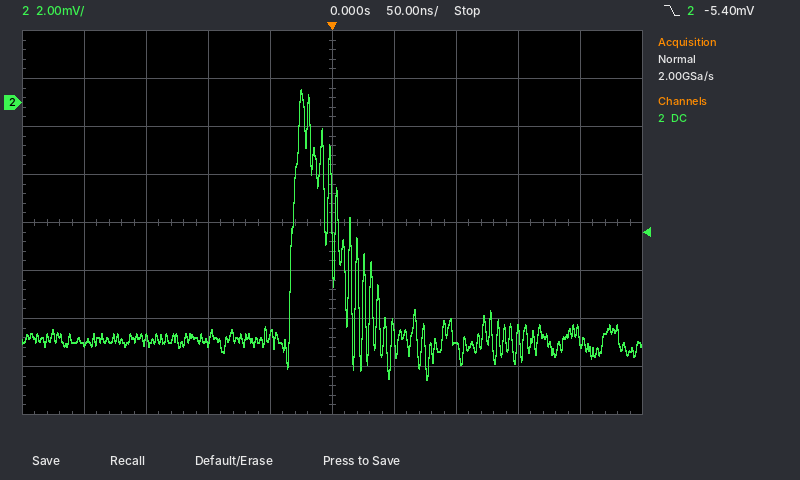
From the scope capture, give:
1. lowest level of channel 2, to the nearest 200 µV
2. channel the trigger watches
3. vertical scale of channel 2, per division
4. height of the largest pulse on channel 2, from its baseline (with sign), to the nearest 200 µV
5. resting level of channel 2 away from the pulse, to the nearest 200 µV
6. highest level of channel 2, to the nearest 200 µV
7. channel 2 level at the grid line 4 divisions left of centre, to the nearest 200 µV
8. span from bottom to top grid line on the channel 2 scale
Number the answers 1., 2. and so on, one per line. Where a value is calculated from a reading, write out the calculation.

1. -11.6 mV
2. channel 2
3. 2 mV
4. 600 µV − (-9.8 mV) = +10.4 mV
5. -9.8 mV
6. 600 µV
7. -10.0 mV
8. 16 mV
